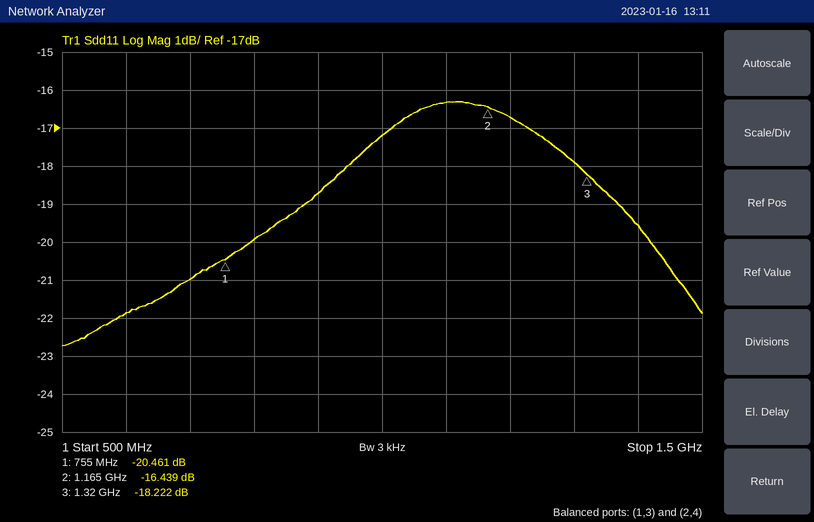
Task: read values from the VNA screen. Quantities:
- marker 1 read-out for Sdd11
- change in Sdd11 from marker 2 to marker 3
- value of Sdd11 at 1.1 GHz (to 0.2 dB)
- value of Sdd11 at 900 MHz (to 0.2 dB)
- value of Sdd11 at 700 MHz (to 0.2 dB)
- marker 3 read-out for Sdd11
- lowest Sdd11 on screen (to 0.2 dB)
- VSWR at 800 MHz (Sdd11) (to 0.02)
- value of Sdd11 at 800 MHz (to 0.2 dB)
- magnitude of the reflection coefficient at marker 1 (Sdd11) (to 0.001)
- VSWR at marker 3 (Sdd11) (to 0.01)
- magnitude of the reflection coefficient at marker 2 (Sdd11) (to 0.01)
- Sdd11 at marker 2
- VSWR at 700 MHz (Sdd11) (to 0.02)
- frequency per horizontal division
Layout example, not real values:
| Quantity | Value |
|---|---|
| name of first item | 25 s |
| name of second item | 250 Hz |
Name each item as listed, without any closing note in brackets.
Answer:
| Quantity | Value |
|---|---|
| marker 1 read-out for Sdd11 | -20.461 dB |
| change in Sdd11 from marker 2 to marker 3 | -1.783 dB |
| value of Sdd11 at 1.1 GHz | -16.4 dB |
| value of Sdd11 at 900 MHz | -18.8 dB |
| value of Sdd11 at 700 MHz | -21.0 dB |
| marker 3 read-out for Sdd11 | -18.222 dB |
| lowest Sdd11 on screen | -22.8 dB |
| VSWR at 800 MHz (Sdd11) | 1.22 |
| value of Sdd11 at 800 MHz | -20.0 dB |
| magnitude of the reflection coefficient at marker 1 (Sdd11) | 0.095 |
| VSWR at marker 3 (Sdd11) | 1.28 |
| magnitude of the reflection coefficient at marker 2 (Sdd11) | 0.15 |
| Sdd11 at marker 2 | -16.439 dB |
| VSWR at 700 MHz (Sdd11) | 1.20 |
| frequency per horizontal division | 100 MHz |
